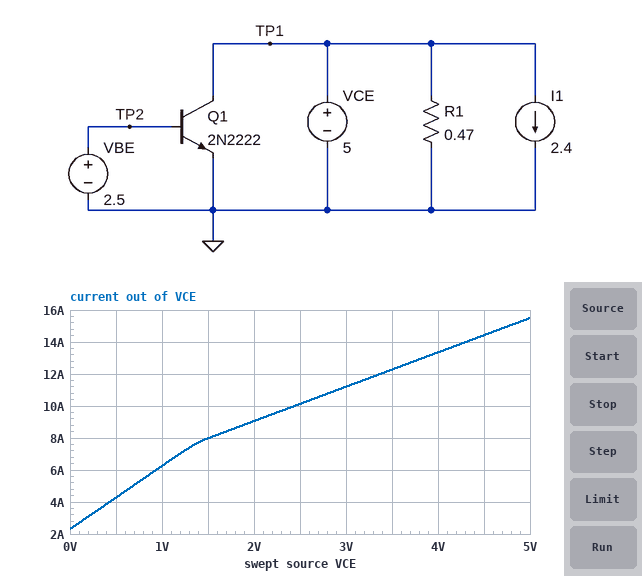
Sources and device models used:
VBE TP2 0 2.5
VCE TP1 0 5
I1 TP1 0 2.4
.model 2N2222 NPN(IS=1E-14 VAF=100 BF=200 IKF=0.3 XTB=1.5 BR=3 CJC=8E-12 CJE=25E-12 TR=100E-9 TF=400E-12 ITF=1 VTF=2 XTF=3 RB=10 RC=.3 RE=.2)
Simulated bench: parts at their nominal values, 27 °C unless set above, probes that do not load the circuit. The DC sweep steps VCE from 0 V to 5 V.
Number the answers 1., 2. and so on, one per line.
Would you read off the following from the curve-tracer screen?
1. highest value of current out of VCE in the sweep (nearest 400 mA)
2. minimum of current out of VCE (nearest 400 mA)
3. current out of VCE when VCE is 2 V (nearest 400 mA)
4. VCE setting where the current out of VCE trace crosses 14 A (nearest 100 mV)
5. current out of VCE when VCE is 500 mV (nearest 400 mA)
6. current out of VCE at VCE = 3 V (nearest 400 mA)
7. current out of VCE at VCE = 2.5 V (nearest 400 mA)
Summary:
1. 15.6 A
2. 2.4 A
3. 9.2 A
4. 4.3 V
5. 4.4 A
6. 11.2 A
7. 10.0 A
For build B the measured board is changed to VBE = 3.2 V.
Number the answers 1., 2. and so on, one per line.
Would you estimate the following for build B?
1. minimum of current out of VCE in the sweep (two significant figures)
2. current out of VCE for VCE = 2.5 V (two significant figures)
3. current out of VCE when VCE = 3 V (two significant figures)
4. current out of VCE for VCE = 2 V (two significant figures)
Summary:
1. 2.3 A
2. 11 A
3. 12 A
4. 9.6 A
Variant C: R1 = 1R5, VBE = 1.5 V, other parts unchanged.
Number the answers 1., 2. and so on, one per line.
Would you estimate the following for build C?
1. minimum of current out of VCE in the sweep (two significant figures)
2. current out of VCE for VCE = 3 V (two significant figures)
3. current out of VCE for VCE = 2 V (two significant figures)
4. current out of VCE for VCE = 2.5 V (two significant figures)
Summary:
1. 2.4 A
2. 5.7 A
3. 5.0 A
4. 5.4 A
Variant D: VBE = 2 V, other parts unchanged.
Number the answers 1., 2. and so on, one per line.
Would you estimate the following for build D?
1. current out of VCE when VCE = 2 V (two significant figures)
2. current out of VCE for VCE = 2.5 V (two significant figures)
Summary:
1. 8.6 A
2. 9.6 A
